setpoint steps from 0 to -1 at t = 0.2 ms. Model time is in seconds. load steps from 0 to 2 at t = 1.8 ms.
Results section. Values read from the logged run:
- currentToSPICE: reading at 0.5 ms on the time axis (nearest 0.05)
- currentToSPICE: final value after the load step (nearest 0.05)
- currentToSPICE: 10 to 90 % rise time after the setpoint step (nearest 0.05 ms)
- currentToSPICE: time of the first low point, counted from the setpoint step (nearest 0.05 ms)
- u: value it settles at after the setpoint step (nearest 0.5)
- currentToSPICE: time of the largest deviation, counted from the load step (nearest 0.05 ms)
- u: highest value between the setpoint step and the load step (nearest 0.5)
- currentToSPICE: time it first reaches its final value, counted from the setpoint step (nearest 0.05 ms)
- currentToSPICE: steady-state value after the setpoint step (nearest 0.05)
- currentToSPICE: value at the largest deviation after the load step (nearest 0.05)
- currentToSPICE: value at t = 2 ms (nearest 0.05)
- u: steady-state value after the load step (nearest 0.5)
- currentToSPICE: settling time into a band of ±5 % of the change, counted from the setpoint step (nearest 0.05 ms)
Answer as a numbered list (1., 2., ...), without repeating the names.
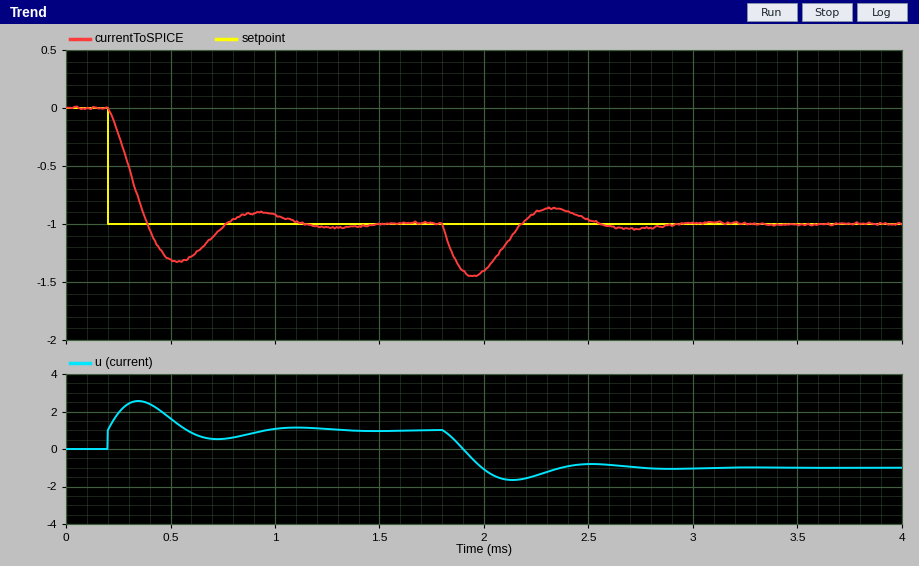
1. -1.30
2. -1.00
3. 0.15 ms
4. 0.35 ms
5. 1.0
6. 0.15 ms
7. 2.5
8. 0.20 ms
9. -1.00
10. -1.45
11. -1.40
12. -1.0
13. 0.85 ms
